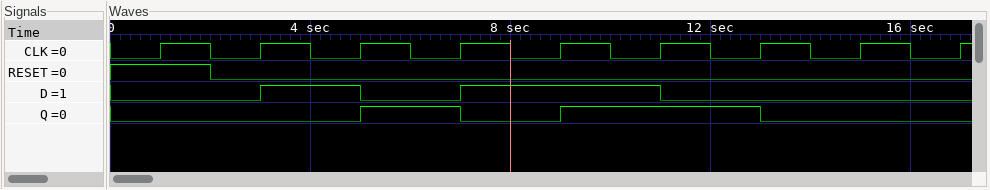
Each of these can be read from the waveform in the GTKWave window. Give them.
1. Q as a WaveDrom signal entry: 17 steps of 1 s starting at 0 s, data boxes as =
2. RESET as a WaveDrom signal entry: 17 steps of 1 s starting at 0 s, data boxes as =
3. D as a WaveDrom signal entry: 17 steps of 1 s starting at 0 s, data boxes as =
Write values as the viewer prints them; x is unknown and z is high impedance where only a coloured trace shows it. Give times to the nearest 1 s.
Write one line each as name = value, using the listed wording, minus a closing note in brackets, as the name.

Q as a WaveDrom signal entry: 17 steps of 1 s starting at 0 s, data boxes as = = {name: 'Q', wave: '0....1.0.1...0...'}
RESET as a WaveDrom signal entry: 17 steps of 1 s starting at 0 s, data boxes as = = {name: 'RESET', wave: '1.0..............'}
D as a WaveDrom signal entry: 17 steps of 1 s starting at 0 s, data boxes as = = {name: 'D', wave: '0..1.0.1...0.....'}
